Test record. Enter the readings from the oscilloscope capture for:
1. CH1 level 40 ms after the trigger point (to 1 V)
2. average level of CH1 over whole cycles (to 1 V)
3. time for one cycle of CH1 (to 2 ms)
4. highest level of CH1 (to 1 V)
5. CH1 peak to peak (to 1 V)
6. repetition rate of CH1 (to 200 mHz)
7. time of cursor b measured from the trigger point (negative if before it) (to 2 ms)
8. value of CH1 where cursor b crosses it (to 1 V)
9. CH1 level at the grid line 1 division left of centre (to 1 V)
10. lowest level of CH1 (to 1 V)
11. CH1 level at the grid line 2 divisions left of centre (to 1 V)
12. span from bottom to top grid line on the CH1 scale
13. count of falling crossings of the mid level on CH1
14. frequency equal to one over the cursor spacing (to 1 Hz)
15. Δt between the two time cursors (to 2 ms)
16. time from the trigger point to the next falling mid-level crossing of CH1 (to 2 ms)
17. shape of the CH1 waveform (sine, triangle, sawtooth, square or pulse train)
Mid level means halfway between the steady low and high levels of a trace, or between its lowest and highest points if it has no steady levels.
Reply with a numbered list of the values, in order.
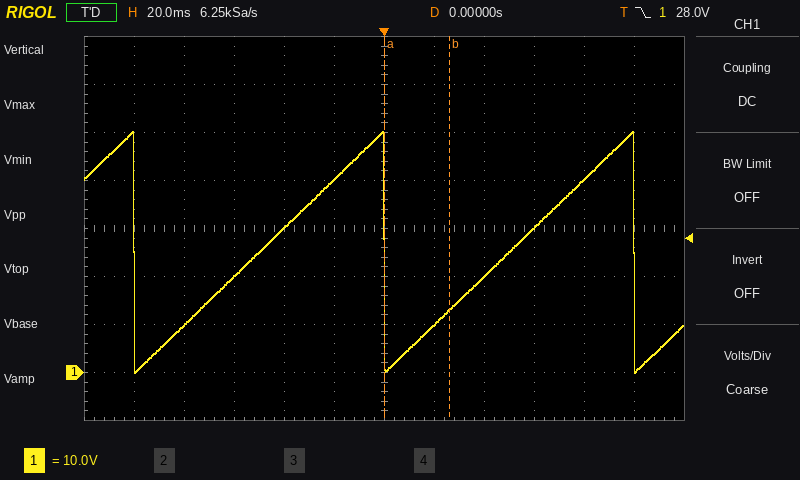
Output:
1. 20 V
2. 25 V
3. 100 ms
4. 50 V
5. 50 V
6. 10.0 Hz
7. +26 ms
8. 13 V
9. 40 V
10. 0 V
11. 30 V
12. 80 V
13. 3
14. 38 Hz
15. 26 ms
16. 100 ms
17. sawtooth
